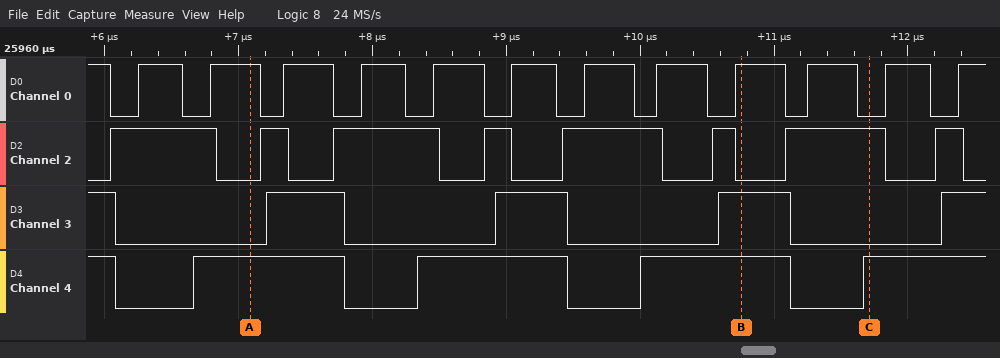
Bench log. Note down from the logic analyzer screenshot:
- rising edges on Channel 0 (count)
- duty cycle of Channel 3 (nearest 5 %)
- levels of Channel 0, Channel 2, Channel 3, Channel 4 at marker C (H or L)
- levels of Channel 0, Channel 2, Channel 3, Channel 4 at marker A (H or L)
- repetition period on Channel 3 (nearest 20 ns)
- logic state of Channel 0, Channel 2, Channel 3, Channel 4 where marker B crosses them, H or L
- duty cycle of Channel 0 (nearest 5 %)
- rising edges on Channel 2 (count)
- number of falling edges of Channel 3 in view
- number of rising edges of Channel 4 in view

12
35 %
Channel 0=L, Channel 2=H, Channel 3=L, Channel 4=H
Channel 0=H, Channel 2=L, Channel 3=L, Channel 4=H
1680 ns
Channel 0=H, Channel 2=L, Channel 3=H, Channel 4=H
65 %
8
4
4
